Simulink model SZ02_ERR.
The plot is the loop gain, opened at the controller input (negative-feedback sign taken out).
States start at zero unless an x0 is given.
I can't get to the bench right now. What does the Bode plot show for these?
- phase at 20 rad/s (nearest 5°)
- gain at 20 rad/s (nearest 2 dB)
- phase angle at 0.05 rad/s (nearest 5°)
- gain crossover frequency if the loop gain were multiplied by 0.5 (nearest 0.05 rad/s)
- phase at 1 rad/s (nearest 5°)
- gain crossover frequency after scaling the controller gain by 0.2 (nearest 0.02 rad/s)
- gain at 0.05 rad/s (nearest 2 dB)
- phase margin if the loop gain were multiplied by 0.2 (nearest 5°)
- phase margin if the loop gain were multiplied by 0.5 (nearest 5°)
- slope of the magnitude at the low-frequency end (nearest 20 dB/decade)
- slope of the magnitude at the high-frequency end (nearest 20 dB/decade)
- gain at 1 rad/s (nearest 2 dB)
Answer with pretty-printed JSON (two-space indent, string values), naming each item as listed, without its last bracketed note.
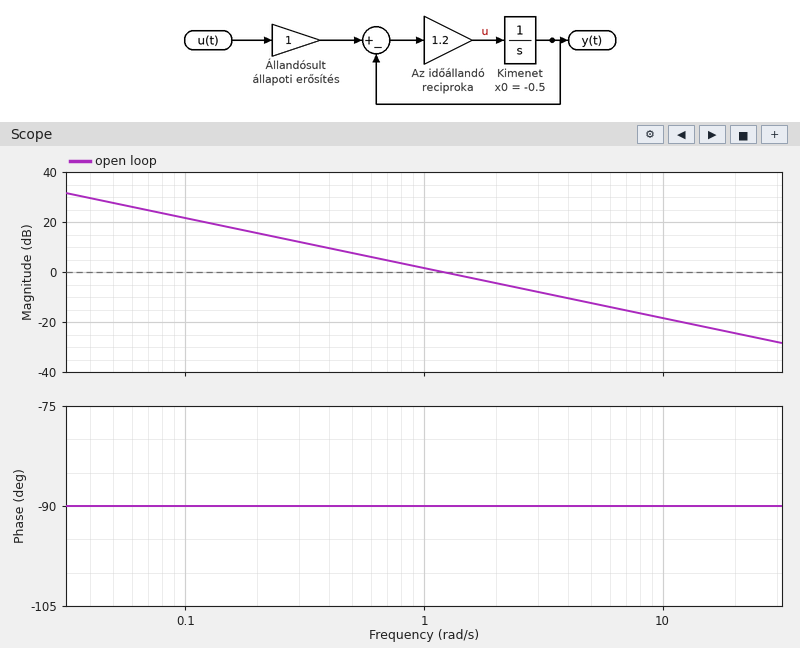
{
  "phase at 20 rad/s": "-90°",
  "gain at 20 rad/s": "-24 dB",
  "phase angle at 0.05 rad/s": "-90°",
  "gain crossover frequency if the loop gain were multiplied by 0.5": "0.60 rad/s",
  "phase at 1 rad/s": "-90°",
  "gain crossover frequency after scaling the controller gain by 0.2": "0.24 rad/s",
  "gain at 0.05 rad/s": "28 dB",
  "phase margin if the loop gain were multiplied by 0.2": "90°",
  "phase margin if the loop gain were multiplied by 0.5": "90°",
  "slope of the magnitude at the low-frequency end": "-20 dB/decade",
  "slope of the magnitude at the high-frequency end": "-20 dB/decade",
  "gain at 1 rad/s": "2 dB"
}
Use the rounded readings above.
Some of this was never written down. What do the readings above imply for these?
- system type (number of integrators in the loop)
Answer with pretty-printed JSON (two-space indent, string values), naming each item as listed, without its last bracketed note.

{
  "system type": "1"
}
